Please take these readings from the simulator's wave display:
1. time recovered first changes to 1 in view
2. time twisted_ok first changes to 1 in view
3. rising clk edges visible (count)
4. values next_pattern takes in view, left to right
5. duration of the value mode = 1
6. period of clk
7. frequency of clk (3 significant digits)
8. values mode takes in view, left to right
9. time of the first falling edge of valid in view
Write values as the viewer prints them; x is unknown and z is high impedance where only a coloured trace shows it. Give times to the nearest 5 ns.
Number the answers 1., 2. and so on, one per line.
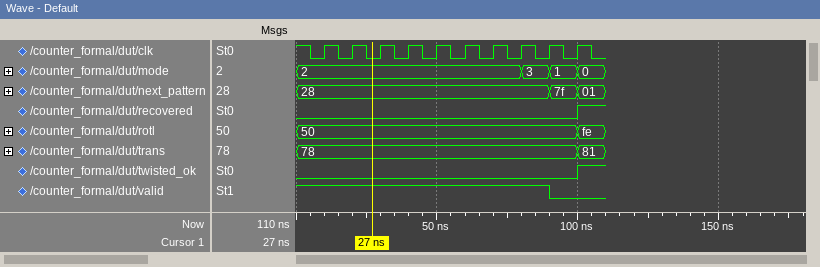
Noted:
1. 100 ns
2. 100 ns
3. 10
4. 28, 7f, 01
5. 10 ns
6. 10 ns
7. 100 MHz
8. 2, 3, 1, 0
9. 90 ns
